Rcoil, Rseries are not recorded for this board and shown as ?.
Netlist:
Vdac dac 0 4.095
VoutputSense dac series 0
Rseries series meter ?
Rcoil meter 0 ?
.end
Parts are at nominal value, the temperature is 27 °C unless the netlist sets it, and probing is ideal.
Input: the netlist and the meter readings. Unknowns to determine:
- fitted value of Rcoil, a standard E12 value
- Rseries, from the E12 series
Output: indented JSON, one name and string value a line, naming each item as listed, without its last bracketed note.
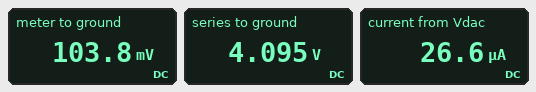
{
  "fitted value of Rcoil, a standard E12 value": "3.9 kΩ",
  "Rseries, from the E12 series": "150 kΩ"
}
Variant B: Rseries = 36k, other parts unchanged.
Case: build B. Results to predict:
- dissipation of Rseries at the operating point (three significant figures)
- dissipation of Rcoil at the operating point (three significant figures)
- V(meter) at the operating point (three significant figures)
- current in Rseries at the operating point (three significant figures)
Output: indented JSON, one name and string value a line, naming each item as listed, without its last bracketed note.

{
  "dissipation of Rseries at the operating point": "379 µW",
  "dissipation of Rcoil at the operating point": "41.1 µW",
  "V(meter) at the operating point": "400 mV",
  "current in Rseries at the operating point": "103 µA"
}
